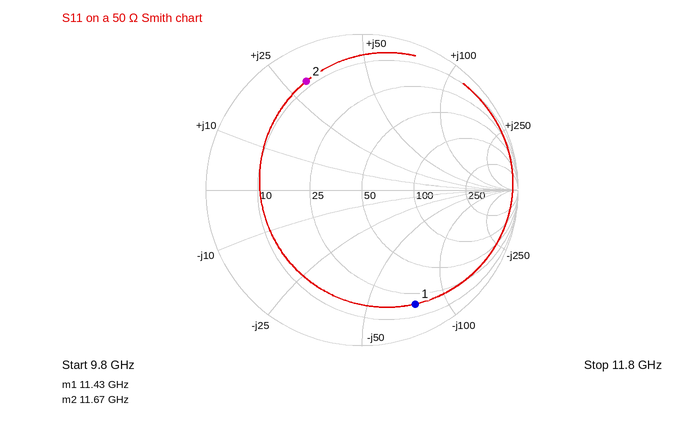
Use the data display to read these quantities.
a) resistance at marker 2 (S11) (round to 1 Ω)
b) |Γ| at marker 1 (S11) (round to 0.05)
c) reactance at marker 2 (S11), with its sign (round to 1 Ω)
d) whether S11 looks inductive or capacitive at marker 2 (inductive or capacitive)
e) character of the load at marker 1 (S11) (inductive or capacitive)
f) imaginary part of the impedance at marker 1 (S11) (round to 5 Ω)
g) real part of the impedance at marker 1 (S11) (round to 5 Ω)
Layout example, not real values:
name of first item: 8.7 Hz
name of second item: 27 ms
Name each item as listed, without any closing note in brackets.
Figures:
resistance at marker 2 (S11): 8 Ω
|Γ| at marker 1 (S11): 0.80
reactance at marker 2 (S11), with its sign: +30 Ω
whether S11 looks inductive or capacitive at marker 2: inductive
character of the load at marker 1 (S11): capacitive
imaginary part of the impedance at marker 1 (S11): -75 Ω
real part of the impedance at marker 1 (S11): 20 Ω
